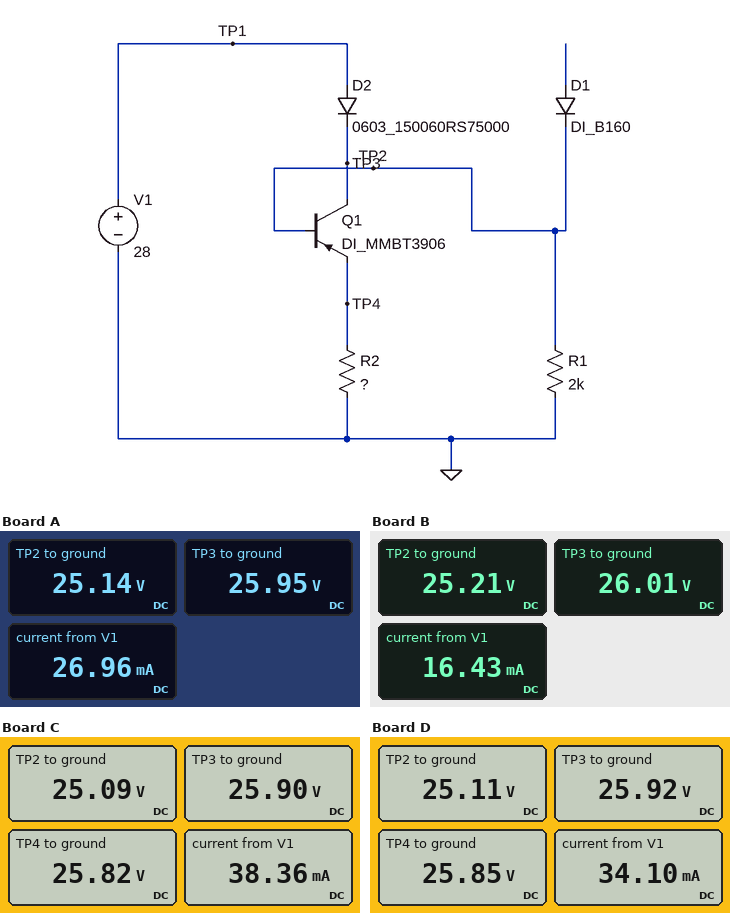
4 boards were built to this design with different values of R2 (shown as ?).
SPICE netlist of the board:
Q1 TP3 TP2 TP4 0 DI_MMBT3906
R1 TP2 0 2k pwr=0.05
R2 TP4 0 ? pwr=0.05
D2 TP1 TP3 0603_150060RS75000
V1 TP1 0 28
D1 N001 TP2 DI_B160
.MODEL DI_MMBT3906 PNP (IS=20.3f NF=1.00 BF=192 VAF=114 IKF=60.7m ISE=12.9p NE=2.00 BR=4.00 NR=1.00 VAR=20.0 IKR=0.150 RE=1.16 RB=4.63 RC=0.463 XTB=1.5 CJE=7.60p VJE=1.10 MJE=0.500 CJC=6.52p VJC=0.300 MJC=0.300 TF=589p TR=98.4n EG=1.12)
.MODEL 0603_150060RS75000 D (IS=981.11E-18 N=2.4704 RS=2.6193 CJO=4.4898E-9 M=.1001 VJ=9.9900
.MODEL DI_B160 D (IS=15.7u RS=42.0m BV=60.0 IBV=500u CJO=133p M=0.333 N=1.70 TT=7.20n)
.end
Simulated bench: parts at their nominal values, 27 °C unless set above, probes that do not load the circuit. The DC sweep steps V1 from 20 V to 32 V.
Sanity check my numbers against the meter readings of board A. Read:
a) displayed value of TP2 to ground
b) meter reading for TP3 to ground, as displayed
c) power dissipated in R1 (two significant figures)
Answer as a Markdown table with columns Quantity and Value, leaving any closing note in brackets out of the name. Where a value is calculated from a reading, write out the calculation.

| Quantity | Value |
|---|---|
| displayed value of TP2 to ground | 25.14 V |
| meter reading for TP3 to ground, as displayed | 25.95 V |
| power dissipated in R1 | (25.14 V)^2 / 2 kΩ = 320 mW |
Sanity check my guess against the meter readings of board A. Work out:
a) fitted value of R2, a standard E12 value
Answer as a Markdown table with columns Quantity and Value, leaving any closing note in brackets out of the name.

| Quantity | Value |
|---|---|
| fitted value of R2, a standard E12 value | 1.8 kΩ |
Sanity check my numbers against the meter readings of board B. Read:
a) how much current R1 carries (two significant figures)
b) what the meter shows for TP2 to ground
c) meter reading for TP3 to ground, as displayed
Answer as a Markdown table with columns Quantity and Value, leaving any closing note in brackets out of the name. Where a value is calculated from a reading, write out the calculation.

| Quantity | Value |
|---|---|
| how much current R1 carries | (25.21 V) / 2 kΩ = 13 mA |
| what the meter shows for TP2 to ground | 25.21 V |
| meter reading for TP3 to ground, as displayed | 26.01 V |
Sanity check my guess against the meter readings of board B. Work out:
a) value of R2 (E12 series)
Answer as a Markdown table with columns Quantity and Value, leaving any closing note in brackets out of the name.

| Quantity | Value |
|---|---|
| value of R2 | 6.8 kΩ |
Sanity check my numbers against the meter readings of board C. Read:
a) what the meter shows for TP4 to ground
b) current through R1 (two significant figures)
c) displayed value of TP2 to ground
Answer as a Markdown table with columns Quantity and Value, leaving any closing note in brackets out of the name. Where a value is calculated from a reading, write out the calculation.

| Quantity | Value |
|---|---|
| what the meter shows for TP4 to ground | 25.82 V |
| current through R1 | (25.09 V) / 2 kΩ = 13 mA |
| displayed value of TP2 to ground | 25.09 V |
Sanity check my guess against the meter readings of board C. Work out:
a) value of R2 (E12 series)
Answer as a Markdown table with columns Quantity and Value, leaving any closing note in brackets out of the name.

| Quantity | Value |
|---|---|
| value of R2 | 1 kΩ |
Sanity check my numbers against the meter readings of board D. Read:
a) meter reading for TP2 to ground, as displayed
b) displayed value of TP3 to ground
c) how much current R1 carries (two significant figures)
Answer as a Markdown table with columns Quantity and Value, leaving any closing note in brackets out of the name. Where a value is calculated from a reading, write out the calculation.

| Quantity | Value |
|---|---|
| meter reading for TP2 to ground, as displayed | 25.11 V |
| displayed value of TP3 to ground | 25.92 V |
| how much current R1 carries | (25.11 V) / 2 kΩ = 13 mA |
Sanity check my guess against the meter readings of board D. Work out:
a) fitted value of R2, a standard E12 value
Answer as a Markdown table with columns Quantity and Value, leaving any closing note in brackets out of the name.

| Quantity | Value |
|---|---|
| fitted value of R2, a standard E12 value | 1.2 kΩ |
